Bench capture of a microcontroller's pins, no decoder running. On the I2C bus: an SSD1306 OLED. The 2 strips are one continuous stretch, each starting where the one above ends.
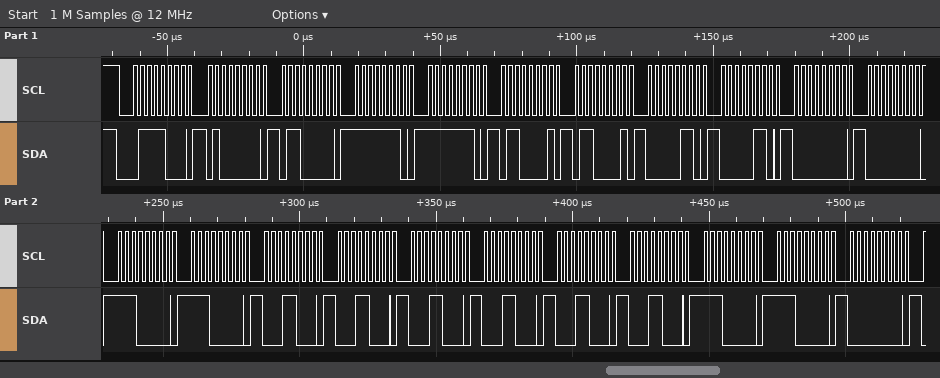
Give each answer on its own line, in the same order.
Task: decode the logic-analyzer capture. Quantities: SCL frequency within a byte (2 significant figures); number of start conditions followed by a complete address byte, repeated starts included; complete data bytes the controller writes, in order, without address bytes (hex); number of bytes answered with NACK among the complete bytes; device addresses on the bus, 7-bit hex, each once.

400 kHz
1
40 60 FE FE 61 61 06 06 00 00 E0 E0 18 18 18 18 18 18 E0 E0 00
0
0x3C
